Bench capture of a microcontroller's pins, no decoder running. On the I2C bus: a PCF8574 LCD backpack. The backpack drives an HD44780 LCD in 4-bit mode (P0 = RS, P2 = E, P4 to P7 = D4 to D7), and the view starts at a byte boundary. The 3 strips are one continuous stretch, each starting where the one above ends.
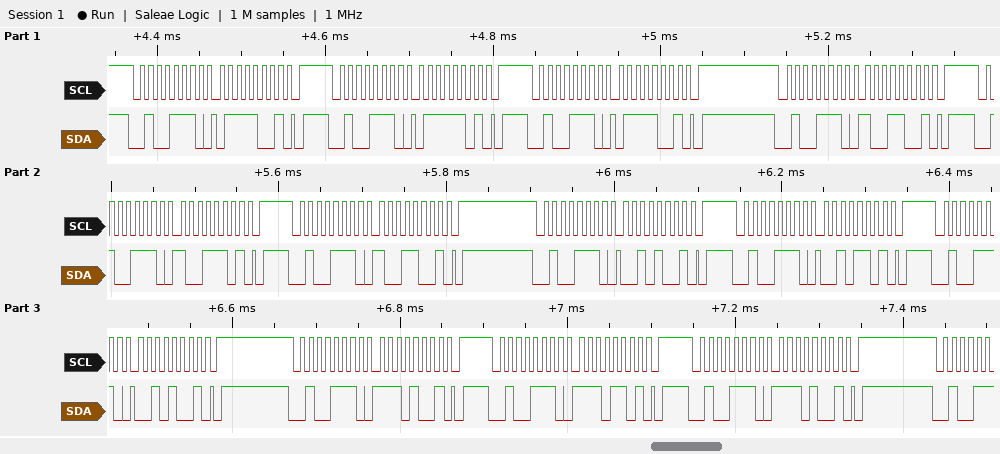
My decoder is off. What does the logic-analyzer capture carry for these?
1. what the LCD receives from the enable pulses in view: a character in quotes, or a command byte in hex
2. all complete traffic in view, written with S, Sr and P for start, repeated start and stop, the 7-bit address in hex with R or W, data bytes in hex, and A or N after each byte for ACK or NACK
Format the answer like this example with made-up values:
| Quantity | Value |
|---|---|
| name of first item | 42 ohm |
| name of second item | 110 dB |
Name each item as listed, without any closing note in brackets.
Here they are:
| Quantity | Value |
|---|---|
| what the LCD receives from the enable pulses in view: a character in quotes, or a command byte in hex | 'y' '.' |
| all complete traffic in view, written with S, Sr and P for start, repeated start and stop, the 7-bit address in hex with R or W, data bytes in hex, and A or N after each byte for ACK or NACK | S 27W A 79 A P S 27W A 7D A P S 27W A 79 A P S 27W A 99 A P S 27W A 9D A P S 27W A 99 A P S 27W A 29 A P S 27W A 2D A P S 27W A 29 A P S 27W A E9 A P S 27W A ED A P S 27W A E9 A P |
